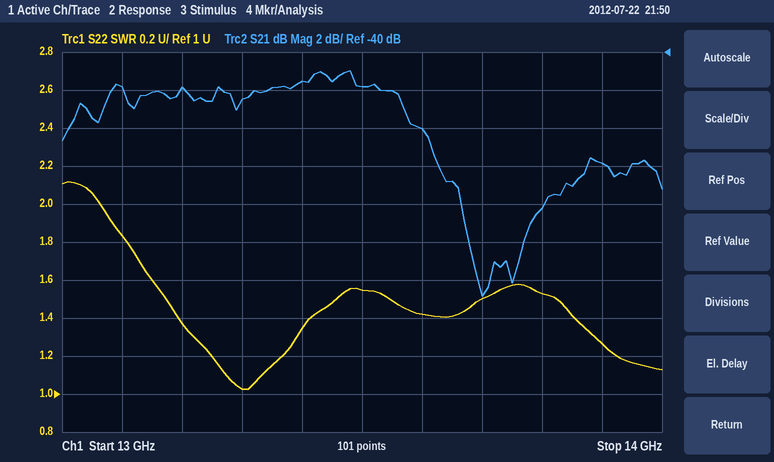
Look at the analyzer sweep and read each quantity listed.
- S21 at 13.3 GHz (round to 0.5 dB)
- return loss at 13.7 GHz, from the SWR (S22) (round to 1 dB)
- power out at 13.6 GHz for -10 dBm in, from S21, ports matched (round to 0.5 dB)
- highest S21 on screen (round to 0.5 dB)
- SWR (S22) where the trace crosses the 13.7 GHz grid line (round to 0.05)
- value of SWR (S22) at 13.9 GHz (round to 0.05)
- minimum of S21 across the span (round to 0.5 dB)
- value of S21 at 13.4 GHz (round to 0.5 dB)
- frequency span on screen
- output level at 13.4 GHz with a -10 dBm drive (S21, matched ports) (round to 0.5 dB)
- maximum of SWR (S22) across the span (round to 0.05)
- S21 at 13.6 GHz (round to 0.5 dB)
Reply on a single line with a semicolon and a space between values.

-42.5 dB; 14 dB; -54.0 dBm; -41.0 dB; 1.50; 1.25; -53.0 dB; -41.5 dB; 1 GHz; -51.5 dBm; 2.10; -44.0 dB
